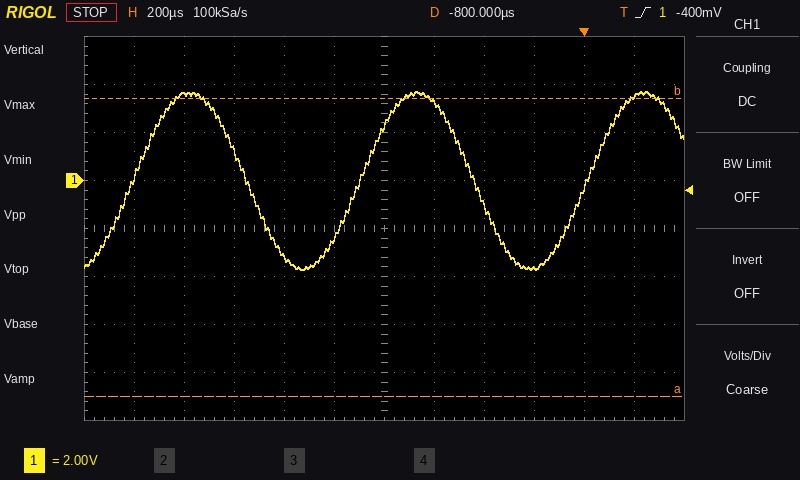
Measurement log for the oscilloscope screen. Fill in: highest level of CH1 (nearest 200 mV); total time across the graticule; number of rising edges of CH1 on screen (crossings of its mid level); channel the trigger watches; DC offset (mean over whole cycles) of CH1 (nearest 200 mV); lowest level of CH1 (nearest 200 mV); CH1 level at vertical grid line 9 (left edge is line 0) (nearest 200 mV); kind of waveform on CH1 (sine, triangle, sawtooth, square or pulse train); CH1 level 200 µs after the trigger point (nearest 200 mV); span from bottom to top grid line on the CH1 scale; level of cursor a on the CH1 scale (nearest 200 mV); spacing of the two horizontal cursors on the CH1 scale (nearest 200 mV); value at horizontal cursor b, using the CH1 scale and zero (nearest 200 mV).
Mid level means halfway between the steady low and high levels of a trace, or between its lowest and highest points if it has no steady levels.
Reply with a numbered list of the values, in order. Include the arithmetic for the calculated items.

1. 3.8 V
2. 2.4 ms
3. 3
4. CH1
5. (3.8 V + (-3.8 V)) / 2 ≈ 0.0 V
6. -3.8 V
7. -3.6 V
8. sine
9. 3.6 V
10. 16 V
11. -9.0 V
12. 12.4 V
13. 3.4 V
